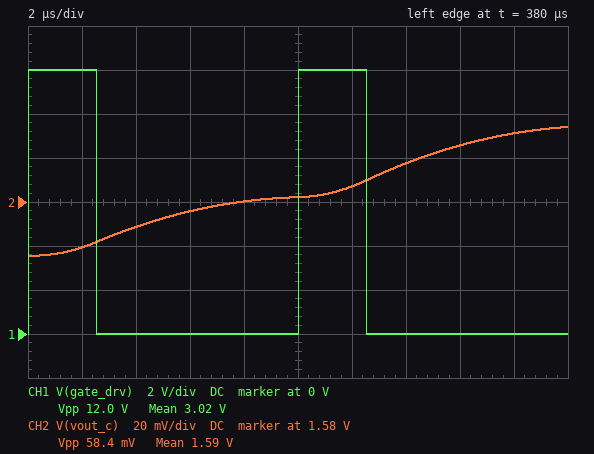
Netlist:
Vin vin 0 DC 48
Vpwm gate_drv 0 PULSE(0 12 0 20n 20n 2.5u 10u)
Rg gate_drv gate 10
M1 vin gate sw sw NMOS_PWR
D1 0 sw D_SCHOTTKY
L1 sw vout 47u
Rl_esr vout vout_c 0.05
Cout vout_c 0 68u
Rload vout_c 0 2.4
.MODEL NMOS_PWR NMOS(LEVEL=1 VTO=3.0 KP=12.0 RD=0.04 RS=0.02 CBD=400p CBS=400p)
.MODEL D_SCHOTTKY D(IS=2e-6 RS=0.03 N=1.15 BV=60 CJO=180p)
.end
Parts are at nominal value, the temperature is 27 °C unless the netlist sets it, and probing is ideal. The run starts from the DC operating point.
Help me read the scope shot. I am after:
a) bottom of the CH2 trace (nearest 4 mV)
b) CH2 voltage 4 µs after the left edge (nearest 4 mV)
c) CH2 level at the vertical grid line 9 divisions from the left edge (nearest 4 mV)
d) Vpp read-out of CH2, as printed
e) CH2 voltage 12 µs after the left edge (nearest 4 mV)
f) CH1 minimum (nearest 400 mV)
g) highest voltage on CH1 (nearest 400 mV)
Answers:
1.556 V
1.568 V
1.612 V
58.4 mV
1.588 V
0 V
12.0 V
